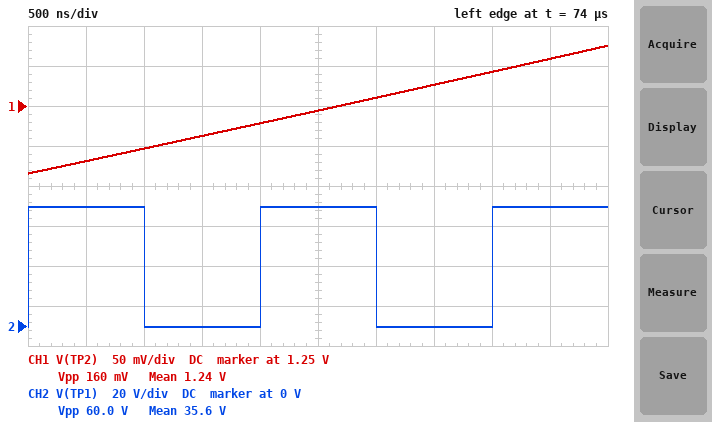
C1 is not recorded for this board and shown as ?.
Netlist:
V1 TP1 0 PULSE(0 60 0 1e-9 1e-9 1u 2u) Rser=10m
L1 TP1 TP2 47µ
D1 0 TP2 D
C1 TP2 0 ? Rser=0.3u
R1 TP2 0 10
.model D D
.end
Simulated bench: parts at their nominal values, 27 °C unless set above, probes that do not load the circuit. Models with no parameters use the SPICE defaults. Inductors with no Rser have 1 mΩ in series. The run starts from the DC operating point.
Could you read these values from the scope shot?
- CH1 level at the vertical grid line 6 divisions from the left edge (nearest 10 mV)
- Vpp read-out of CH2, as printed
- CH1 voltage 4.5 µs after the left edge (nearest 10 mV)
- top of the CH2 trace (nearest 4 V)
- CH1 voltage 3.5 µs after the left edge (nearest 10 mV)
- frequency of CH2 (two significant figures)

1.26 V
60.0 V
1.31 V
60 V
1.28 V
500 kHz
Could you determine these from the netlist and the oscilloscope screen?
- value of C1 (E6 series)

1.5 mF
